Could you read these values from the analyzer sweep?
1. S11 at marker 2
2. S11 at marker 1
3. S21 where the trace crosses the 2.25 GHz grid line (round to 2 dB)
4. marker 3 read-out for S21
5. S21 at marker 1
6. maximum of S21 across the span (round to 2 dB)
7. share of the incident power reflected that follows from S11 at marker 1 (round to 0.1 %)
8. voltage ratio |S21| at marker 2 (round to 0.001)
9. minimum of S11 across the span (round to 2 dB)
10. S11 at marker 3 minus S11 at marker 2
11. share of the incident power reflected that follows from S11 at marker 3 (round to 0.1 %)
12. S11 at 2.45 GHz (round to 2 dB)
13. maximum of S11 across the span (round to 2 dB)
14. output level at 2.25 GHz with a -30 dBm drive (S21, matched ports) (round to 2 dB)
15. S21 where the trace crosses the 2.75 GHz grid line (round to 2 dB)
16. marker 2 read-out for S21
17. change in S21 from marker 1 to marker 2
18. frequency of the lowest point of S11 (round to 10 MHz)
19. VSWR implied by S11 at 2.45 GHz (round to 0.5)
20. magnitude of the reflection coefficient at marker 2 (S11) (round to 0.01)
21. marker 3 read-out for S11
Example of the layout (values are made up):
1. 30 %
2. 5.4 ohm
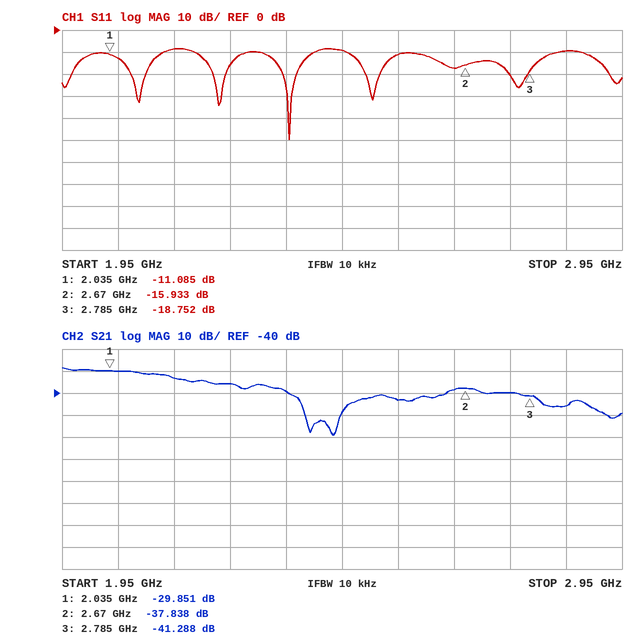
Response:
1. -15.933 dB
2. -11.085 dB
3. -36 dB
4. -41.288 dB
5. -29.851 dB
6. -28 dB
7. 7.8 %
8. 0.013
9. -50 dB
10. -2.819 dB
11. 1.3 %
12. -10 dB
13. -8 dB
14. -66 dBm
15. -40 dB
16. -37.838 dB
17. -7.987 dB
18. 2.36 GHz
19. 2.0
20. 0.16
21. -18.752 dB
